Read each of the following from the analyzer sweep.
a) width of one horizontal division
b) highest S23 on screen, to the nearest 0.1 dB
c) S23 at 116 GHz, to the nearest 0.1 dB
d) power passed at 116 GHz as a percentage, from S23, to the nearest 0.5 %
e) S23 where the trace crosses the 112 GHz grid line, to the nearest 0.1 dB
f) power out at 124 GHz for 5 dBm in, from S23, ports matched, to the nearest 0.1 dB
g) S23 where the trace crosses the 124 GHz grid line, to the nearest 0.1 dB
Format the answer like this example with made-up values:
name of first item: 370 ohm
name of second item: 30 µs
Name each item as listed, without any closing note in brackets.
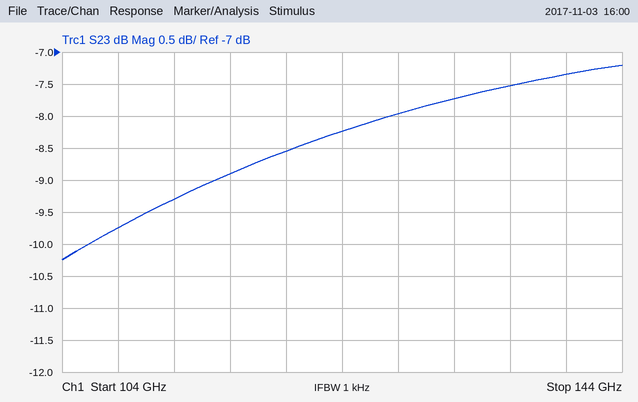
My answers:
width of one horizontal division: 4 GHz
highest S23 on screen, to the nearest 0.1 dB: -7.2 dB
S23 at 116 GHz, to the nearest 0.1 dB: -8.9 dB
power passed at 116 GHz as a percentage, from S23, to the nearest 0.5 %: 13.0 %
S23 where the trace crosses the 112 GHz grid line, to the nearest 0.1 dB: -9.3 dB
power out at 124 GHz for 5 dBm in, from S23, ports matched, to the nearest 0.1 dB: -3.2 dBm
S23 where the trace crosses the 124 GHz grid line, to the nearest 0.1 dB: -8.2 dB
